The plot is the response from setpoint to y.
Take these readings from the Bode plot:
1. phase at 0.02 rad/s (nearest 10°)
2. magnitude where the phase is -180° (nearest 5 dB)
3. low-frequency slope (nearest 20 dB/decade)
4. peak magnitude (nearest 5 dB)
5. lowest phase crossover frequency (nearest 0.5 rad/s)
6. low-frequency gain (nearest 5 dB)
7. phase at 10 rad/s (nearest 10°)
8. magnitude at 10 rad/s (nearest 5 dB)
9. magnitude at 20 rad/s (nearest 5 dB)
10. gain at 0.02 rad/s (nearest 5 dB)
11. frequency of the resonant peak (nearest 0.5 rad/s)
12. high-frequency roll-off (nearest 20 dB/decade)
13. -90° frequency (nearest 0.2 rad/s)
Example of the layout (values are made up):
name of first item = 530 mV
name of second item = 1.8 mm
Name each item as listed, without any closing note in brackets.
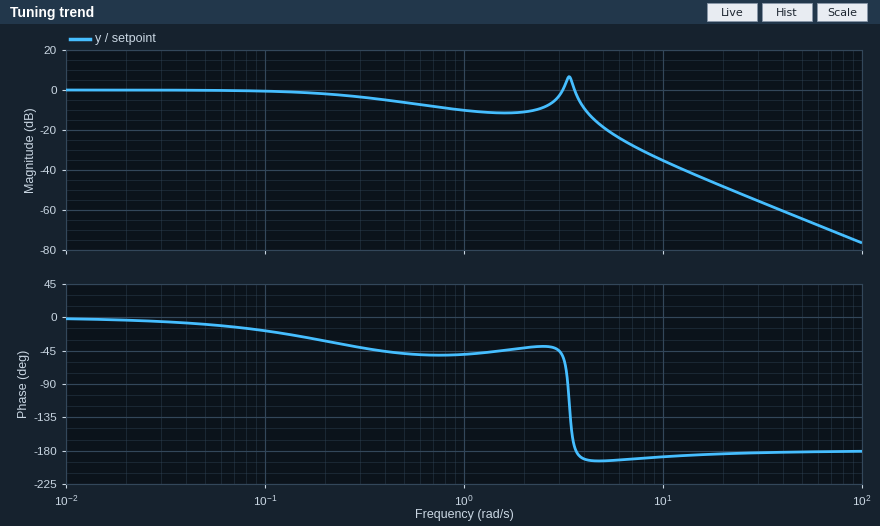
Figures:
phase at 0.02 rad/s = 0°
magnitude where the phase is -180° = 0 dB
low-frequency slope = 0 dB/decade
peak magnitude = 5 dB
lowest phase crossover frequency = 3.5 rad/s
low-frequency gain = 0 dB
phase at 10 rad/s = -190°
magnitude at 10 rad/s = -35 dB
magnitude at 20 rad/s = -50 dB
gain at 0.02 rad/s = 0 dB
frequency of the resonant peak = 3.5 rad/s
high-frequency roll-off = -40 dB/decade
-90° frequency = 3.4 rad/s
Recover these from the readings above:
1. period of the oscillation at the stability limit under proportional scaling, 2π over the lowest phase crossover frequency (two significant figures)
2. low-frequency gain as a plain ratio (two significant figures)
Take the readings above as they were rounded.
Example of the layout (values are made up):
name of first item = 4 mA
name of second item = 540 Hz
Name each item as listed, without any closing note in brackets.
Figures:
period of the oscillation at the stability limit under proportional scaling, 2π over the lowest phase crossover frequency = 1.8 s
low-frequency gain as a plain ratio = 1.0
